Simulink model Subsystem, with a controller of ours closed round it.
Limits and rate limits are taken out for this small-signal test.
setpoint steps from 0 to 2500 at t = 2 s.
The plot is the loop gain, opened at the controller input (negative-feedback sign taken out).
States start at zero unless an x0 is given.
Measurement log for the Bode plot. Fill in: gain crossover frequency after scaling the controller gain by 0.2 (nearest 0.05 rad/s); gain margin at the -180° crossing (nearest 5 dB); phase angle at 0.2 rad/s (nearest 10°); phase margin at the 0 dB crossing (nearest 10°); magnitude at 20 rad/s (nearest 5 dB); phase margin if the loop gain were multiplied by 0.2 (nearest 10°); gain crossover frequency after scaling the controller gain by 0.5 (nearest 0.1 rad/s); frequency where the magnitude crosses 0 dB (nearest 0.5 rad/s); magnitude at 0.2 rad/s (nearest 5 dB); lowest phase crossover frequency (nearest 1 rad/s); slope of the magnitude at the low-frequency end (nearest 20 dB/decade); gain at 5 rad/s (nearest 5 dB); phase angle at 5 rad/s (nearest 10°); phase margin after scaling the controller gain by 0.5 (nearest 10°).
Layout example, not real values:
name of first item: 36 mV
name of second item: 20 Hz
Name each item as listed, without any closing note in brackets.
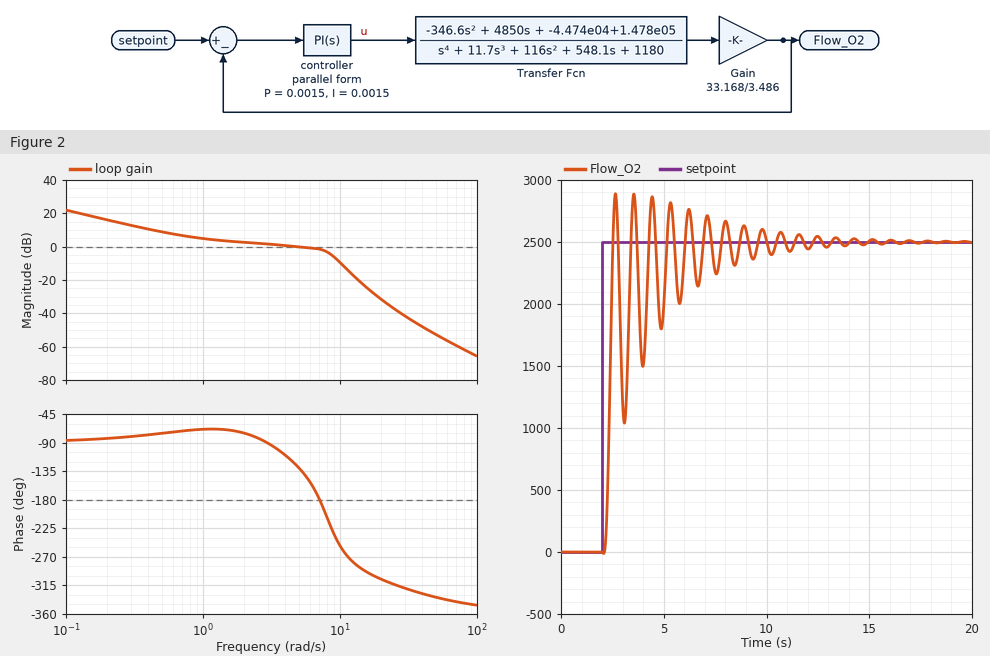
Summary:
gain crossover frequency after scaling the controller gain by 0.2: 0.25 rad/s
gain margin at the -180° crossing: 0 dB
phase angle at 0.2 rad/s: -80°
phase margin at the 0 dB crossing: 50°
magnitude at 20 rad/s: -30 dB
phase margin if the loop gain were multiplied by 0.2: 100°
gain crossover frequency after scaling the controller gain by 0.5: 0.8 rad/s
frequency where the magnitude crosses 0 dB: 5.0 rad/s
magnitude at 0.2 rad/s: 15 dB
lowest phase crossover frequency: 7 rad/s
slope of the magnitude at the low-frequency end: -20 dB/decade
gain at 5 rad/s: 0 dB
phase angle at 5 rad/s: -130°
phase margin after scaling the controller gain by 0.5: 110°
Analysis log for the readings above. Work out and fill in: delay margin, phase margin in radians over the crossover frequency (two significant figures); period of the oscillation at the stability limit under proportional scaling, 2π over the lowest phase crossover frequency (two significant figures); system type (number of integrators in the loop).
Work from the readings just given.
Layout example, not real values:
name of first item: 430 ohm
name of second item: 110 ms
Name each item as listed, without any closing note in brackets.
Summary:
delay margin, phase margin in radians over the crossover frequency: 0.17 s
period of the oscillation at the stability limit under proportional scaling, 2π over the lowest phase crossover frequency: 0.90 s
system type: 1
